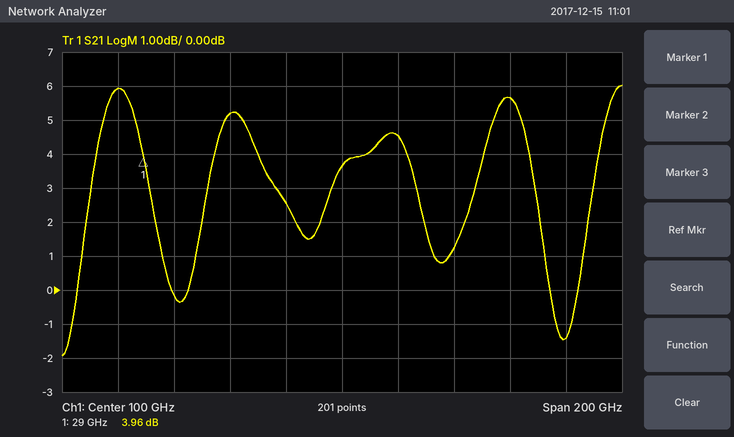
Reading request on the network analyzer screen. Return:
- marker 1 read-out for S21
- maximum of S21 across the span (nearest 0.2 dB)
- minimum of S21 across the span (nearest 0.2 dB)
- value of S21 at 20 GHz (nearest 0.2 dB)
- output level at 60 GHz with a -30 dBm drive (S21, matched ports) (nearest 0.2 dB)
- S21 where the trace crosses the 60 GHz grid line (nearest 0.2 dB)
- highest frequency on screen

3.96 dB
6.0 dB
-2.0 dB
6.0 dB
-24.8 dBm
5.2 dB
200 GHz
